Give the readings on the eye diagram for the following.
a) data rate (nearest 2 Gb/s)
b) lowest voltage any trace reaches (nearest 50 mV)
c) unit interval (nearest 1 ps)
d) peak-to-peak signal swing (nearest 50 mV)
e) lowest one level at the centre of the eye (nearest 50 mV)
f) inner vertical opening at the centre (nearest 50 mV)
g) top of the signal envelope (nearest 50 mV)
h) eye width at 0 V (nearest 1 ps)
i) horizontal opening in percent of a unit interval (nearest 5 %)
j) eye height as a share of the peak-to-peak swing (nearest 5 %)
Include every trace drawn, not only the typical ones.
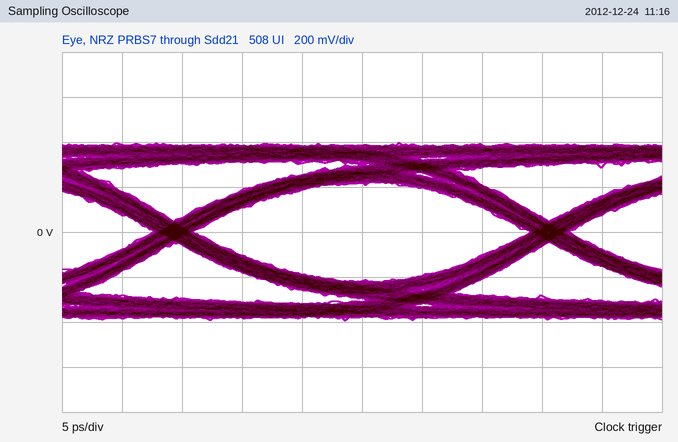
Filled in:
32 Gb/s
-400 mV
31 ps
800 mV
200 mV
450 mV
400 mV
28 ps
90 %
55 %
